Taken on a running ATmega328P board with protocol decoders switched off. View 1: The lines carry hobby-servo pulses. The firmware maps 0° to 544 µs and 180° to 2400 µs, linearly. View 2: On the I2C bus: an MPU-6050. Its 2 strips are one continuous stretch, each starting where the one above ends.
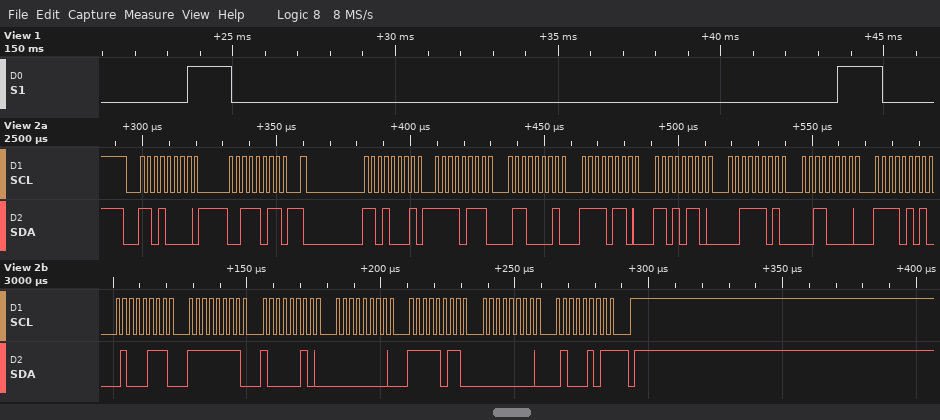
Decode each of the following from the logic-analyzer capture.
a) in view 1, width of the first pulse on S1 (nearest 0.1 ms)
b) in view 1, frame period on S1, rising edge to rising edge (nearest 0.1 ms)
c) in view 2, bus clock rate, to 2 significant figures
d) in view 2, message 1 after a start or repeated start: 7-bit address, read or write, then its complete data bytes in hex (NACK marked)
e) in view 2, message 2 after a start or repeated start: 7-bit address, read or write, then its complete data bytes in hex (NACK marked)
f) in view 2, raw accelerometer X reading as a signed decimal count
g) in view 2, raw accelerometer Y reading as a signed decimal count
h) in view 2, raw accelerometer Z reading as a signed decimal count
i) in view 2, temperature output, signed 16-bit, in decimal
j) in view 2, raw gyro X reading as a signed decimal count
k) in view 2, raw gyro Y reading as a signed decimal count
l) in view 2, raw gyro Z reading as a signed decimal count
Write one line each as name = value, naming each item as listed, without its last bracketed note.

in view 1, width of the first pulse on S1 = 1.4 ms
in view 1, frame period on S1, rising edge to rising edge = 20.0 ms
in view 2, bus clock rate, to 2 significant figures = 400 kHz
in view 2, message 1 after a start or repeated start: 7-bit address, read or write, then its complete data bytes in hex = 0x68 write: 3B
in view 2, message 2 after a start or repeated start: 7-bit address, read or write, then its complete data bytes in hex = 0x68 read: F7 61 F6 D6 3D 30 F5 47 FF 82 00 FB 00 45 NACK
in view 2, raw accelerometer X reading as a signed decimal count = -2207
in view 2, raw accelerometer Y reading as a signed decimal count = -2346
in view 2, raw accelerometer Z reading as a signed decimal count = 15664
in view 2, temperature output, signed 16-bit, in decimal = -2745
in view 2, raw gyro X reading as a signed decimal count = -126
in view 2, raw gyro Y reading as a signed decimal count = 251
in view 2, raw gyro Z reading as a signed decimal count = 69
